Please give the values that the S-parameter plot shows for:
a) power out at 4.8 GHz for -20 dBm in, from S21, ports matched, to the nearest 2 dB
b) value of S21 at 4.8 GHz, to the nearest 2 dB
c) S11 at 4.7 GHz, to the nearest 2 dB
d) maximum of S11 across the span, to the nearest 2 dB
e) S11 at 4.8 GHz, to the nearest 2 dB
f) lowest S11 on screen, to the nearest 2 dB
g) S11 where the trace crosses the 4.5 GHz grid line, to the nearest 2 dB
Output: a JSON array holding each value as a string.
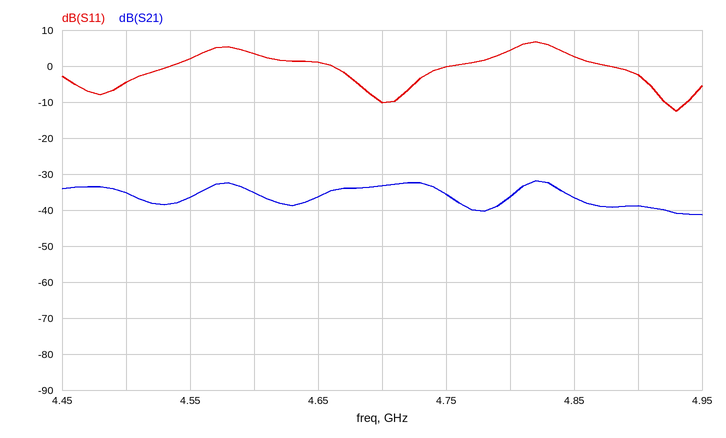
["-56 dBm", "-36 dB", "-10 dB", "6 dB", "4 dB", "-12 dB", "-4 dB"]
